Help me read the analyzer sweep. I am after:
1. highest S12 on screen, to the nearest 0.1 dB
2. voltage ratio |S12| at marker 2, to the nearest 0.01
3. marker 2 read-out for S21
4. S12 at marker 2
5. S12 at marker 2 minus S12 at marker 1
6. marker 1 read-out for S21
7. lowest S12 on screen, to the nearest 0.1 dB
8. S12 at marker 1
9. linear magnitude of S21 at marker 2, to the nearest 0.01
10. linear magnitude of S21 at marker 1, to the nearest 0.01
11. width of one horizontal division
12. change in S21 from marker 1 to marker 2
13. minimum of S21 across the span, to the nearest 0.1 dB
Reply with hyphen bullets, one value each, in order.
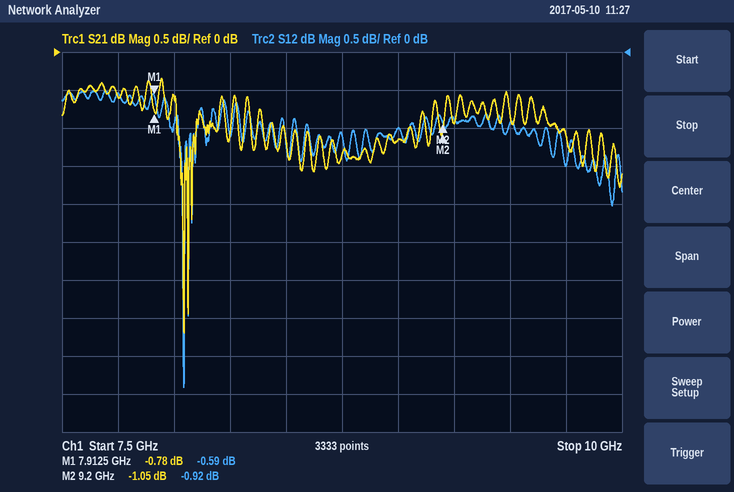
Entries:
- -0.5 dB
- 0.90
- -1.05 dB
- -0.92 dB
- -0.33 dB
- -0.78 dB
- -4.4 dB
- -0.59 dB
- 0.89
- 0.91
- 250 MHz
- -0.27 dB
- -3.7 dB
